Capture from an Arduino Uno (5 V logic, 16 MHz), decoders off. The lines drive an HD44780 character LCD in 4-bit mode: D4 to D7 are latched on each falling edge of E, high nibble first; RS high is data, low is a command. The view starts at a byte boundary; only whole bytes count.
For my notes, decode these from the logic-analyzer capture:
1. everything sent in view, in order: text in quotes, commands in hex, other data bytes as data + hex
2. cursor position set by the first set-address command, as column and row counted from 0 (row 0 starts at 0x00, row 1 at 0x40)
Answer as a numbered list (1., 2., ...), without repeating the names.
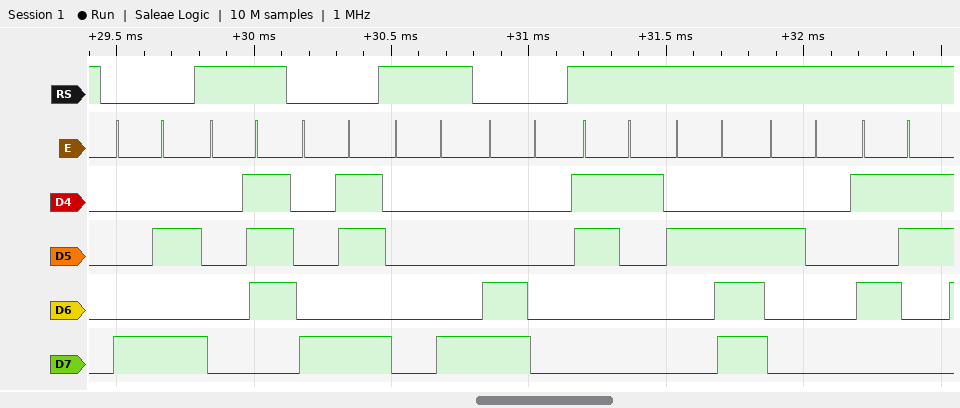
1. 0x8A data 07 0x8B data 08 0xC0 "1. S"
2. column 10, row 0
